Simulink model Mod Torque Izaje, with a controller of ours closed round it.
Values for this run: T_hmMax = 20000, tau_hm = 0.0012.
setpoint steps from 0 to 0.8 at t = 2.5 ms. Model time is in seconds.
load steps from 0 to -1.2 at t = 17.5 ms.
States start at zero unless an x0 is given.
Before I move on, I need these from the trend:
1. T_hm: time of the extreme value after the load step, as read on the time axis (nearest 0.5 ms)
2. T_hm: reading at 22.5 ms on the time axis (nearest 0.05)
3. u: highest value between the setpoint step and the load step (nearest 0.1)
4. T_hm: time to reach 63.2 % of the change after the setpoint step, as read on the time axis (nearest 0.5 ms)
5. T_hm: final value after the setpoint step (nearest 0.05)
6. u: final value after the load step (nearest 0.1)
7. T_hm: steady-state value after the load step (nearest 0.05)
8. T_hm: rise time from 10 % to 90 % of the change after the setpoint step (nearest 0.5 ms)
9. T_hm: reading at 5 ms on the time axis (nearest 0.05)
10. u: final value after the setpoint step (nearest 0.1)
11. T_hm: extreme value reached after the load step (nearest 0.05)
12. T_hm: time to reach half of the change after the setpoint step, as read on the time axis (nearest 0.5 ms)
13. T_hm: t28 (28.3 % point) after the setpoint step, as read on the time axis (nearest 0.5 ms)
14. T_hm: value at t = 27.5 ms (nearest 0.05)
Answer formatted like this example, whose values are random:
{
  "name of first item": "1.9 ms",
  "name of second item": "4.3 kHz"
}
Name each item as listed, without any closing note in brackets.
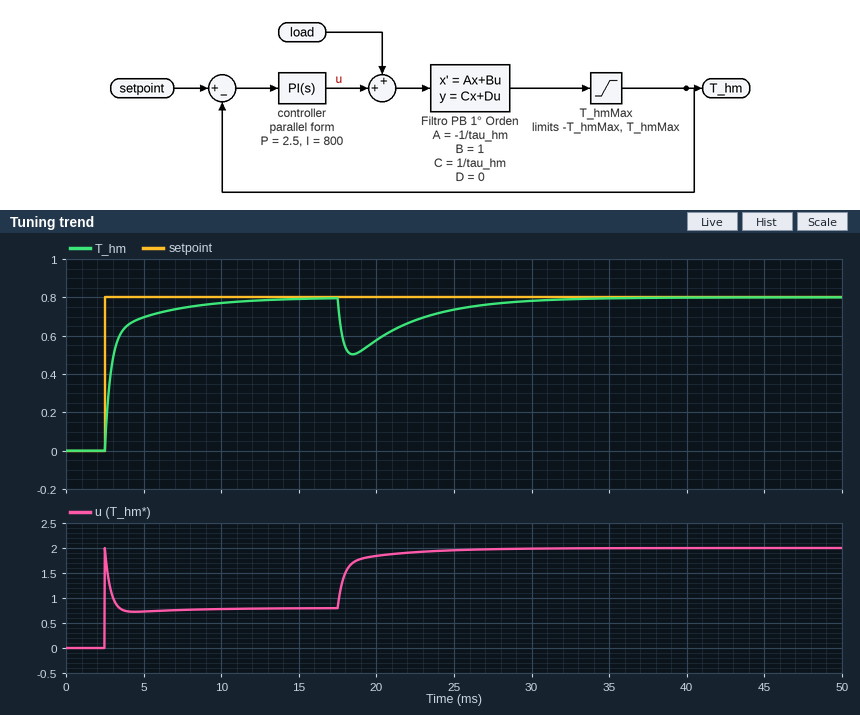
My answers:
{
  "T_hm: time of the extreme value after the load step, as read on the time axis": "18.5 ms",
  "T_hm: reading at 22.5 ms on the time axis": "0.70",
  "u: highest value between the setpoint step and the load step": "2.0",
  "T_hm: time to reach 63.2 % of the change after the setpoint step, as read on the time axis": "3.0 ms",
  "T_hm: final value after the setpoint step": "0.80",
  "u: final value after the load step": "2.0",
  "T_hm: steady-state value after the load step": "0.80",
  "T_hm: rise time from 10 % to 90 % of the change after the setpoint step": "3.5 ms",
  "T_hm: reading at 5 ms on the time axis": "0.70",
  "u: final value after the setpoint step": "0.8",
  "T_hm: extreme value reached after the load step": "0.50",
  "T_hm: time to reach half of the change after the setpoint step, as read on the time axis": "3.0 ms",
  "T_hm: t28 (28.3 % point) after the setpoint step, as read on the time axis": "2.5 ms",
  "T_hm: value at t = 27.5 ms": "0.75"
}
